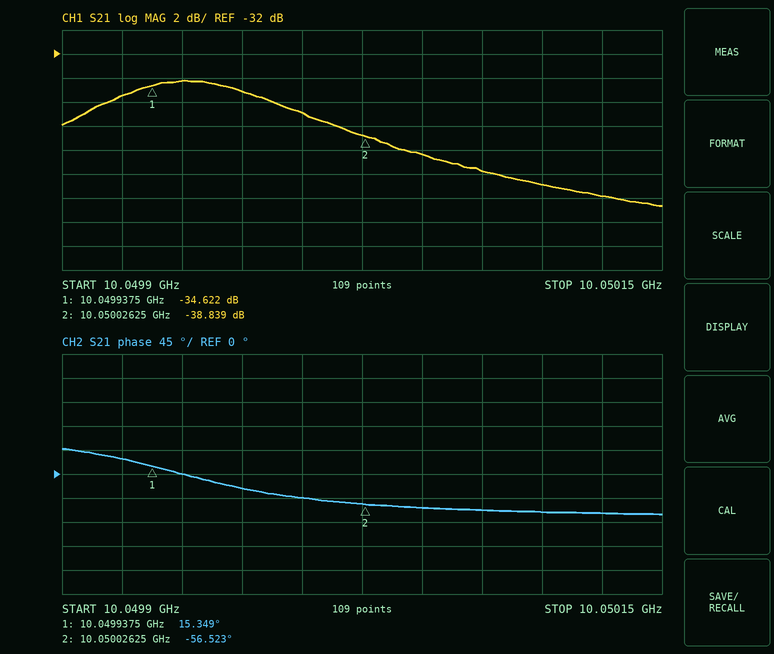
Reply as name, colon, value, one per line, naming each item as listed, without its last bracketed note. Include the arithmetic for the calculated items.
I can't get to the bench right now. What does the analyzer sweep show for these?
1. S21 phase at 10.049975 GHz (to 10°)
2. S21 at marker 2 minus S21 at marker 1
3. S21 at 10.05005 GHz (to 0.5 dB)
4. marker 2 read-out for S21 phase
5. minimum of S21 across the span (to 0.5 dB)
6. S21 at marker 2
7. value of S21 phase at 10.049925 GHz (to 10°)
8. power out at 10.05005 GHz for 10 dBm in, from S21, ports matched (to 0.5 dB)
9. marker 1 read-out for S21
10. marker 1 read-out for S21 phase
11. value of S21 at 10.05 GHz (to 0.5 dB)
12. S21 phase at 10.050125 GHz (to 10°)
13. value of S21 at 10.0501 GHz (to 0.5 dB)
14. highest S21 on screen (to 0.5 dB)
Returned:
S21 phase at 10.049975 GHz: -30°
S21 at marker 2 minus S21 at marker 1: -38.839 − (-34.622) = -4.217 dB
S21 at 10.05005 GHz: -40.5 dB
marker 2 read-out for S21 phase: -56.523°
minimum of S21 across the span: -44.5 dB
S21 at marker 2: -38.839 dB
value of S21 phase at 10.049925 GHz: 30°
power out at 10.05005 GHz for 10 dBm in, from S21, ports matched: 10 dBm + (-40.5 dB) = -30.5 dBm
marker 1 read-out for S21: -34.622 dB
marker 1 read-out for S21 phase: 15.349°
value of S21 at 10.05 GHz: -37.0 dB
S21 phase at 10.050125 GHz: -70°
value of S21 at 10.0501 GHz: -43.0 dB
highest S21 on screen: -34.0 dB
